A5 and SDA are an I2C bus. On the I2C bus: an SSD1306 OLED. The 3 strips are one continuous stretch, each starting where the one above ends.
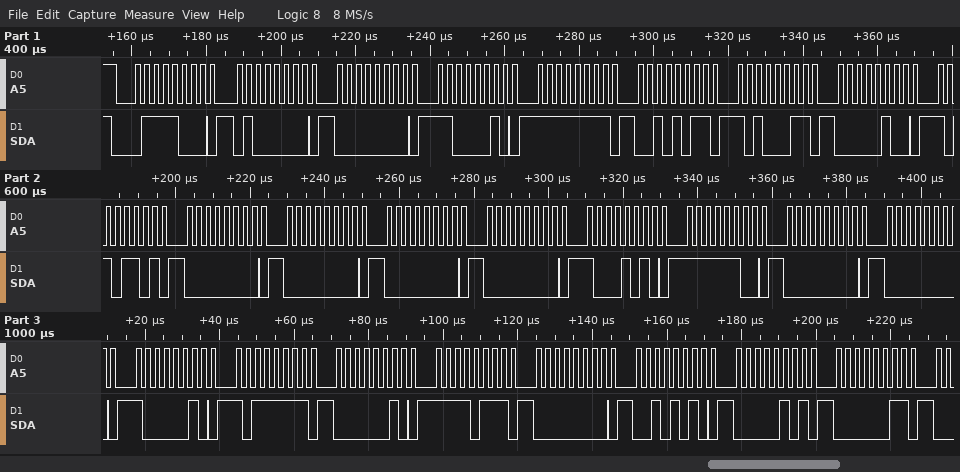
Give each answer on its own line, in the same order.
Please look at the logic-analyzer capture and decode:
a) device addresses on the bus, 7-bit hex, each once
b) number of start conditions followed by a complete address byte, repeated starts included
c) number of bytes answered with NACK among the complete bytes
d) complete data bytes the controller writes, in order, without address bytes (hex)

0x3C
1
0
40 00 C2 FF 2B A3 04 AD 00 00 00 00 8A FC 00 00 82 BF 02 F7 00 2A 05 03
